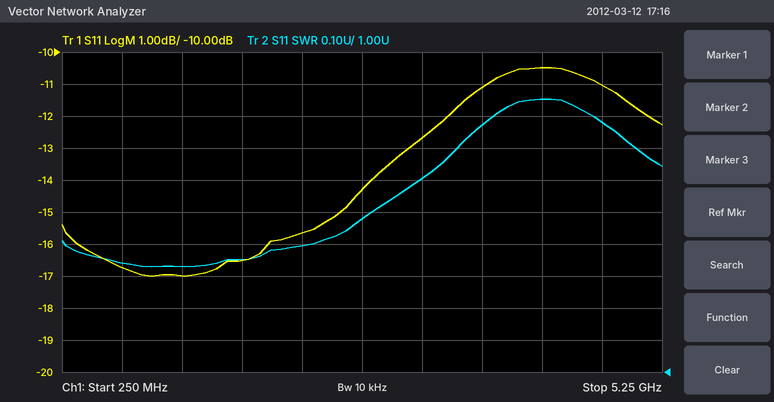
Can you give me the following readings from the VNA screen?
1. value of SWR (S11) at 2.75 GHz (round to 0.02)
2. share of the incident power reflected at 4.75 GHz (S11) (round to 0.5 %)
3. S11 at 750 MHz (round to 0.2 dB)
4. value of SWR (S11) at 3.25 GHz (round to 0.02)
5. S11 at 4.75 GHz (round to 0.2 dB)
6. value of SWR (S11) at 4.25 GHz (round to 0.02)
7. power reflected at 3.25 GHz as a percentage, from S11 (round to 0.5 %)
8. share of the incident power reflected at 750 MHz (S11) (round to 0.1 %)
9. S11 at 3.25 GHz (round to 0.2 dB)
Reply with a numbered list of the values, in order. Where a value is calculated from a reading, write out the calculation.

1. 1.48
2. 10^(-11/10) ≈ 7.94 %, so 8.0 % to the nearest 0.5 %
3. -16.8 dB
4. 1.60
5. -11.0 dB
6. 1.86
7. 10^(-12.6/10) ≈ 5.5 %
8. 10^(-16.8/10) ≈ 2.1 %
9. -12.6 dB
